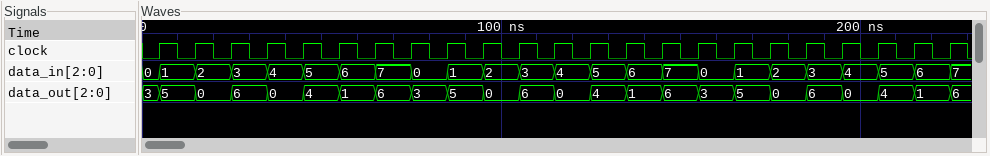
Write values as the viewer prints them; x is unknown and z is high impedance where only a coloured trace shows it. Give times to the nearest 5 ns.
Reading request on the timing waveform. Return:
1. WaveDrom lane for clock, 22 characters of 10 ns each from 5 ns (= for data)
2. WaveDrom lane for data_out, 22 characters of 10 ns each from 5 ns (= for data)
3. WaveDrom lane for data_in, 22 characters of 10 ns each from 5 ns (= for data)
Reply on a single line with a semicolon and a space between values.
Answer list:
{name: 'clock', wave: 'p.....................'}; {name: 'data_out', wave: '======================', data: '5 0 6 0 4 1 6 3 5 0 6 0 4 1 6 3 5 0 6 0 4 1'}; {name: 'data_in', wave: '======================', data: '1 2 3 4 5 6 7 0 1 2 3 4 5 6 7 0 1 2 3 4 5 6'}
